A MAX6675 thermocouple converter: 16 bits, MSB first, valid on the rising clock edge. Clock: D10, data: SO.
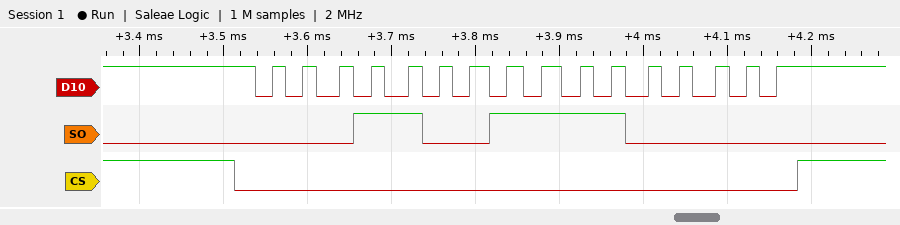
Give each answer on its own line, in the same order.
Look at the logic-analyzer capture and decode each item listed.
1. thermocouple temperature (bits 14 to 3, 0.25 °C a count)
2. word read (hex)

207.00 °C
0x19E0
